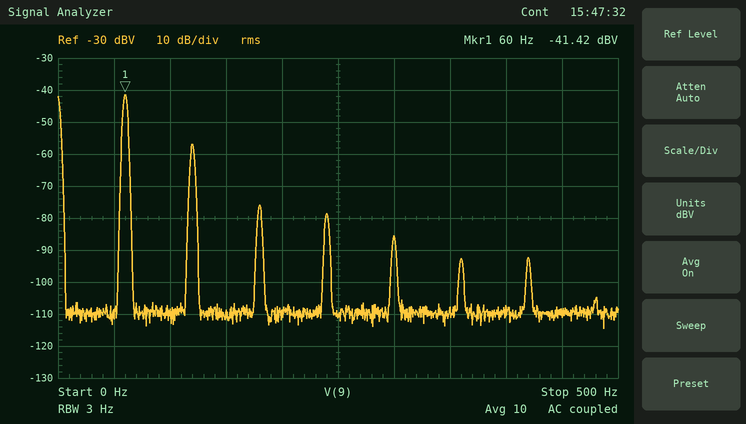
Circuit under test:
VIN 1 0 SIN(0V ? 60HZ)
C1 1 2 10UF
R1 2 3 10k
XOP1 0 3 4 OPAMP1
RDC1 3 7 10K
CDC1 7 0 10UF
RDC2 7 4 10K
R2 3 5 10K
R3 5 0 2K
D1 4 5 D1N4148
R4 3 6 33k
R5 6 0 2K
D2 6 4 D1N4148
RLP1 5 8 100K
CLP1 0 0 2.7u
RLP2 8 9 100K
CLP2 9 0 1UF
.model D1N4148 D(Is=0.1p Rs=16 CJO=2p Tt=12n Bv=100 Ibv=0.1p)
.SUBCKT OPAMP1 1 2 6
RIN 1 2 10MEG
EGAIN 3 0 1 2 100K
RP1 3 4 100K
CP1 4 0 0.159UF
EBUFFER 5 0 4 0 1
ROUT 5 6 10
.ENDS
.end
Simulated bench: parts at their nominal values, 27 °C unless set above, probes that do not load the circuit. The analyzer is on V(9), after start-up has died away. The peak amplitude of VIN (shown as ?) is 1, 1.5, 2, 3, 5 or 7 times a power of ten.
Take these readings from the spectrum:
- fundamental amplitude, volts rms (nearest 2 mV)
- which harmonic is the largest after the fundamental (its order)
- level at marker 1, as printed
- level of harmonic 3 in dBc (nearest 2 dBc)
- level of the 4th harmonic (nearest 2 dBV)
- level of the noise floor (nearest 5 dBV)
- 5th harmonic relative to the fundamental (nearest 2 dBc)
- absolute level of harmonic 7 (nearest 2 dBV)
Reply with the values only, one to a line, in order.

8 mV
2
-41.42 dBV
-34 dBc
-78 dBV
-110 dBV
-44 dBc
-92 dBV
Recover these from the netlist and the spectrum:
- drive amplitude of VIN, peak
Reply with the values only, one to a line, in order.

1.5 V
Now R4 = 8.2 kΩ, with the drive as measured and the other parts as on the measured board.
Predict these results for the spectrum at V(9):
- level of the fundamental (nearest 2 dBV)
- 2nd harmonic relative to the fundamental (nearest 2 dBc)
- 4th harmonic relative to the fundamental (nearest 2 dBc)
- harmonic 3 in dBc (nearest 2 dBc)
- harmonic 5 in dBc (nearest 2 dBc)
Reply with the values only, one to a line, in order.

-44 dBV
-14 dBc
-34 dBc
-50 dBc
-60 dBc
